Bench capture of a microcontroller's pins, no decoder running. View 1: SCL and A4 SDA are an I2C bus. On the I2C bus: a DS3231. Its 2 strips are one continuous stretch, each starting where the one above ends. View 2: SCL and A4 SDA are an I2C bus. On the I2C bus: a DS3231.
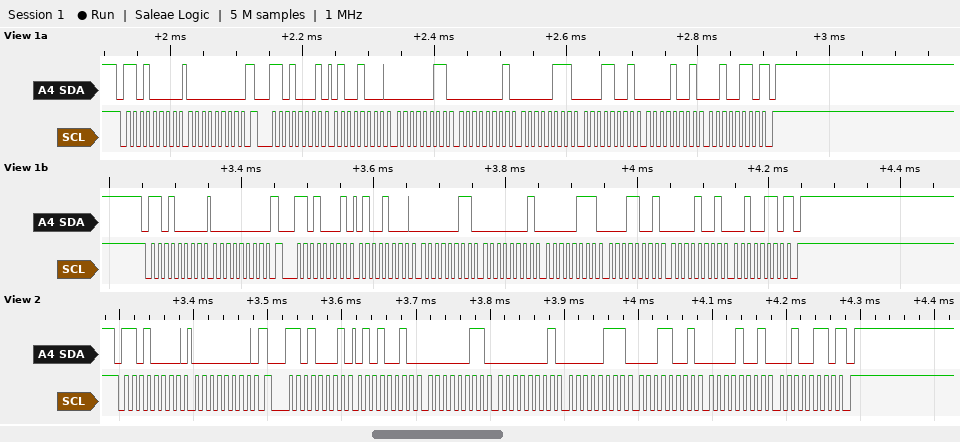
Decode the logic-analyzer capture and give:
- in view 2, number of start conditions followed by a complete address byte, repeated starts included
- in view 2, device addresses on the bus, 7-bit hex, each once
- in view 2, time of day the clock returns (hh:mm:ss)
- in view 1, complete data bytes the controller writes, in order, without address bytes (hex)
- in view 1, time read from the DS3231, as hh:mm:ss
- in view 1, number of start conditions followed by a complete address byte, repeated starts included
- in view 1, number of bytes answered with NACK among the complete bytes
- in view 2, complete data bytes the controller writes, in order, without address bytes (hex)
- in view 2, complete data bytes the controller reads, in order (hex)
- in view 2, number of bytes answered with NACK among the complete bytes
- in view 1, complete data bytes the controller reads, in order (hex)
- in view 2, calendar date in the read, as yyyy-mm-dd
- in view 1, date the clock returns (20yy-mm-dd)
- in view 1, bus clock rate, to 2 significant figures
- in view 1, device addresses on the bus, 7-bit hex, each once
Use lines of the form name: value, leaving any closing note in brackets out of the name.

in view 2, number of start conditions followed by a complete address byte, repeated starts included: 2
in view 2, device addresses on the bus, 7-bit hex, each once: 0x68
in view 2, time of day the clock returns: 01:03:52
in view 1, complete data bytes the controller writes, in order, without address bytes: 00 00
in view 1, time read from the DS3231, as hh:mm:ss: 01:03:48
in view 1, number of start conditions followed by a complete address byte, repeated starts included: 4
in view 1, number of bytes answered with NACK among the complete bytes: 2
in view 2, complete data bytes the controller writes, in order, without address bytes: 00
in view 2, complete data bytes the controller reads, in order: 52 03 01 07 19 09 26
in view 2, number of bytes answered with NACK among the complete bytes: 1
in view 1, complete data bytes the controller reads, in order: 48 03 01 07 19 09 26 48 03 01 07 19 09 26
in view 2, calendar date in the read, as yyyy-mm-dd: 2026-09-19
in view 1, date the clock returns: 2026-09-19
in view 1, bus clock rate, to 2 significant figures: 100 kHz
in view 1, device addresses on the bus, 7-bit hex, each once: 0x68
